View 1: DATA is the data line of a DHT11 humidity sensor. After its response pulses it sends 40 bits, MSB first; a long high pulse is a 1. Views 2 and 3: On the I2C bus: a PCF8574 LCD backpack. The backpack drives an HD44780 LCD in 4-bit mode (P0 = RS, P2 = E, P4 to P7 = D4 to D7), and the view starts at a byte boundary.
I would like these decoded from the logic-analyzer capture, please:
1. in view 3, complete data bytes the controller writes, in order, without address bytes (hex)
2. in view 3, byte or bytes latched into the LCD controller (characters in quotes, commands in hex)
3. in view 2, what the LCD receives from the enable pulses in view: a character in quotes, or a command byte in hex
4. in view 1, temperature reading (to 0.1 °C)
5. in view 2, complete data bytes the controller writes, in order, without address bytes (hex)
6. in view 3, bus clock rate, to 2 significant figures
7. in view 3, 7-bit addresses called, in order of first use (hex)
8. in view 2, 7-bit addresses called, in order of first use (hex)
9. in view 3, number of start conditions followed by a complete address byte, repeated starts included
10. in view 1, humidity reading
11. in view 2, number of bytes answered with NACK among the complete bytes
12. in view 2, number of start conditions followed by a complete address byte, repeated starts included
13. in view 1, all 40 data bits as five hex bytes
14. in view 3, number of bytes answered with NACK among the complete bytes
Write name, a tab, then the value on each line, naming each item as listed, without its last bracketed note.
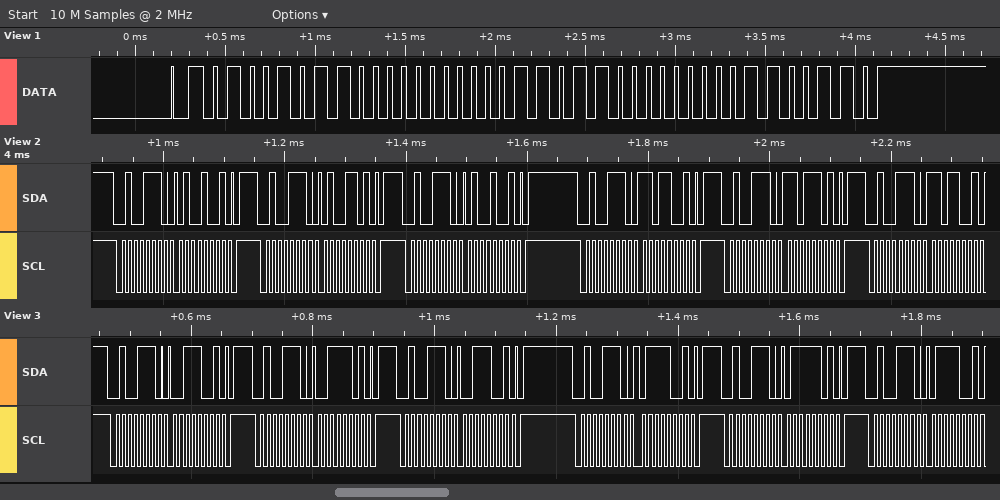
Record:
in view 3, complete data bytes the controller writes, in order, without address bytes	39 3D 39 79 7D 79
in view 3, byte or bytes latched into the LCD controller	'7'
in view 2, what the LCD receives from the enable pulses in view: a character in quotes, or a command byte in hex	'M'
in view 1, temperature reading	27.0 °C
in view 2, complete data bytes the controller writes, in order, without address bytes	49 4D 49 D9 DD D9
in view 3, bus clock rate, to 2 significant figures	100 kHz
in view 3, 7-bit addresses called, in order of first use	0x27
in view 2, 7-bit addresses called, in order of first use	0x27
in view 3, number of start conditions followed by a complete address byte, repeated starts included	6
in view 1, humidity reading	75 %
in view 2, number of bytes answered with NACK among the complete bytes	0
in view 2, number of start conditions followed by a complete address byte, repeated starts included	6
in view 1, all 40 data bits as five hex bytes	4B 00 1B 00 66
in view 3, number of bytes answered with NACK among the complete bytes	0
